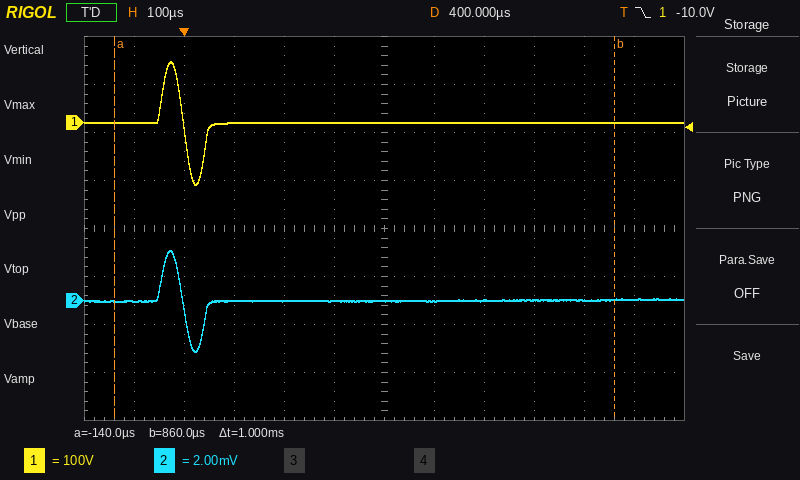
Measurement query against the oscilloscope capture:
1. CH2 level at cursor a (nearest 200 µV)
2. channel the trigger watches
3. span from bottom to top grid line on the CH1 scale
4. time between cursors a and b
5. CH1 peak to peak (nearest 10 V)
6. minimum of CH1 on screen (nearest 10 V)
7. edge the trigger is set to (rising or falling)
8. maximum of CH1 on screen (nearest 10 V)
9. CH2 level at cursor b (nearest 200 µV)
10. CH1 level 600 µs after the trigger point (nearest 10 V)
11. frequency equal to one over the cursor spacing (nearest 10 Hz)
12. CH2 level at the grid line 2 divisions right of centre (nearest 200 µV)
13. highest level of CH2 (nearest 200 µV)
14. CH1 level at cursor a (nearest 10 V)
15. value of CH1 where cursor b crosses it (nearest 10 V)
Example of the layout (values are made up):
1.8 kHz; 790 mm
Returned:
0.0 mV; CH1; 800 V; 1 ms; 260 V; -130 V; falling; 130 V; 0.0 mV; 0 V; 1.00 kHz; 0.0 mV; 2.0 mV; 0 V; 0 V
